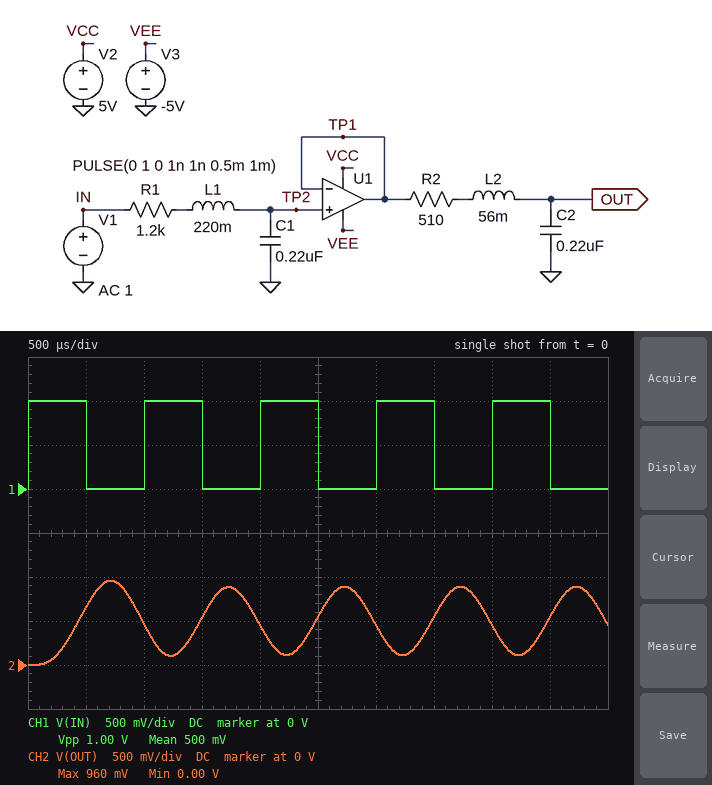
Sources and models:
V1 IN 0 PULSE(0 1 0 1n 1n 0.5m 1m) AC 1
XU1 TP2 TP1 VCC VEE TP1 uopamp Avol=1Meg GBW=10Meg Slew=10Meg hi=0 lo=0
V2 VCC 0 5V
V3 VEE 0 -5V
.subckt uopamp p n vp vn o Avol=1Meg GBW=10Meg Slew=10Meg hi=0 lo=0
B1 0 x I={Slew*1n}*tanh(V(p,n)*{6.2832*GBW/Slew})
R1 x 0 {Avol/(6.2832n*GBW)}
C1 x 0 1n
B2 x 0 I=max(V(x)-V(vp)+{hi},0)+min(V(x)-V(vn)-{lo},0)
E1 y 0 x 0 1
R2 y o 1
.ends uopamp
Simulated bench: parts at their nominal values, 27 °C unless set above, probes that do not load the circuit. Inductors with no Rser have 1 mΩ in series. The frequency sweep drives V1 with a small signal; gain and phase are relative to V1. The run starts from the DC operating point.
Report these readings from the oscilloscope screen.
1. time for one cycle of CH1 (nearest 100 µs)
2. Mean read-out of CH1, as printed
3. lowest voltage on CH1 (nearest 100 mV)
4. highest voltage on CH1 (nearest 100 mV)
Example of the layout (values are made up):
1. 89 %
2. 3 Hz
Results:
1. 1.0 ms
2. 500 mV
3. 0 V
4. 1.0 V
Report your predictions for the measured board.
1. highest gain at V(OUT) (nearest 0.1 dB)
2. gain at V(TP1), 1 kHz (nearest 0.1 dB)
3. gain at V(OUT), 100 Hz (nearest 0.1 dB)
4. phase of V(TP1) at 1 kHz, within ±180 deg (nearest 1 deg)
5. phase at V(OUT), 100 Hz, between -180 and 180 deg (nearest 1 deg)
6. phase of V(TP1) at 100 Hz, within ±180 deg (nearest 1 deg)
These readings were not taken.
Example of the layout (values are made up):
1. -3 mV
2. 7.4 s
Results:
1. 0.7 dB
2. -5.5 dB
3. 0.1 dB
4. -119 deg
5. -14 deg
6. -10 deg
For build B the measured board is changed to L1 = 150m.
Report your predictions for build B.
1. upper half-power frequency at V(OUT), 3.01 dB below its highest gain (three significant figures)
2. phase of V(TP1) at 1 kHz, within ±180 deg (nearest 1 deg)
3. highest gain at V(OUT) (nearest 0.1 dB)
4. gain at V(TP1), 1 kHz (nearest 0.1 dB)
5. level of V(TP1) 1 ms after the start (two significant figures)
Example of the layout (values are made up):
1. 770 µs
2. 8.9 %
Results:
1. 961 Hz
2. -100 deg
3. 0.1 dB
4. -4.5 dB
5. 120 mV
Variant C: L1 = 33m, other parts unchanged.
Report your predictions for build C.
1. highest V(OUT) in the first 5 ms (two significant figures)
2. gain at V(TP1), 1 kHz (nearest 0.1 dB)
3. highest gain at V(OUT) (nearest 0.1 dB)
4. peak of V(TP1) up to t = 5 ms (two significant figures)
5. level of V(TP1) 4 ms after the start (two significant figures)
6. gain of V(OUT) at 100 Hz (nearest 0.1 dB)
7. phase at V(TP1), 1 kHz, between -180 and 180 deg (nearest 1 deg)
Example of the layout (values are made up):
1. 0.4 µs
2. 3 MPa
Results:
1. 910 mV
2. -5.1 dB
3. 0 dB
4. 880 mV
5. 120 mV
6. -0.1 dB
7. -67 deg
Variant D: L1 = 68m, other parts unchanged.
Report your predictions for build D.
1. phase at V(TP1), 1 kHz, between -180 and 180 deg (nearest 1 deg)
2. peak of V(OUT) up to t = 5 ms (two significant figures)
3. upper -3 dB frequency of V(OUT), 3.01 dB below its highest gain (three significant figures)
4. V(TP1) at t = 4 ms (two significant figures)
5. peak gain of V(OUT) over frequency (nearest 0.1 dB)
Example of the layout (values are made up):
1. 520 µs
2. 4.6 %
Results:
1. -76 deg
2. 930 mV
3. 928 Hz
4. 110 mV
5. 0 dB
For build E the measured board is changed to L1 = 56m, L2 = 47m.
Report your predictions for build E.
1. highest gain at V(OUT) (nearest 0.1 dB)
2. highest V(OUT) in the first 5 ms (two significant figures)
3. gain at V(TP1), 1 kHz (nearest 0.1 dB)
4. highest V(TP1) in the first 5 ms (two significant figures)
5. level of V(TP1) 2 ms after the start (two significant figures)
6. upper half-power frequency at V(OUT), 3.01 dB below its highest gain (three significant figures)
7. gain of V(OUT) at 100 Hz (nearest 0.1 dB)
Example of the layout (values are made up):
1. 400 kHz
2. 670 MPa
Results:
1. 0 dB
2. 900 mV
3. -4.8 dB
4. 890 mV
5. 110 mV
6. 827 Hz
7. -0.1 dB
